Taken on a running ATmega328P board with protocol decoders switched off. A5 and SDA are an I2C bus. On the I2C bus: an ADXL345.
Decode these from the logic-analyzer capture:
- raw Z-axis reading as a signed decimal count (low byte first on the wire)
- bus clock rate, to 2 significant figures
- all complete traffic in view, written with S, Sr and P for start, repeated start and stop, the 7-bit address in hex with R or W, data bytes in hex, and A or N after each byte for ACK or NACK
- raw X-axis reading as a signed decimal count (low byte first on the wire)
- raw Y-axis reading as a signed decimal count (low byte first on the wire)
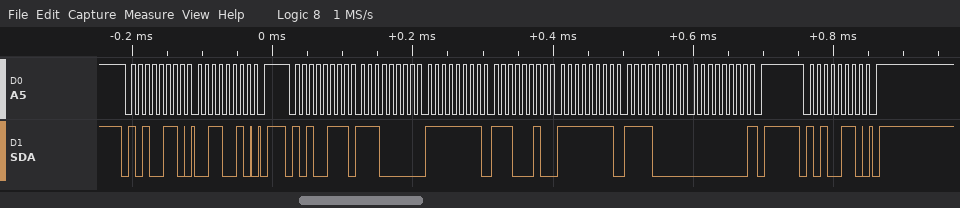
240
100 kHz
S 53W A 32 A P S 53R A E0 A FF A E2 A FF A F0 A 00 N P S 53W A P
-32
-30
